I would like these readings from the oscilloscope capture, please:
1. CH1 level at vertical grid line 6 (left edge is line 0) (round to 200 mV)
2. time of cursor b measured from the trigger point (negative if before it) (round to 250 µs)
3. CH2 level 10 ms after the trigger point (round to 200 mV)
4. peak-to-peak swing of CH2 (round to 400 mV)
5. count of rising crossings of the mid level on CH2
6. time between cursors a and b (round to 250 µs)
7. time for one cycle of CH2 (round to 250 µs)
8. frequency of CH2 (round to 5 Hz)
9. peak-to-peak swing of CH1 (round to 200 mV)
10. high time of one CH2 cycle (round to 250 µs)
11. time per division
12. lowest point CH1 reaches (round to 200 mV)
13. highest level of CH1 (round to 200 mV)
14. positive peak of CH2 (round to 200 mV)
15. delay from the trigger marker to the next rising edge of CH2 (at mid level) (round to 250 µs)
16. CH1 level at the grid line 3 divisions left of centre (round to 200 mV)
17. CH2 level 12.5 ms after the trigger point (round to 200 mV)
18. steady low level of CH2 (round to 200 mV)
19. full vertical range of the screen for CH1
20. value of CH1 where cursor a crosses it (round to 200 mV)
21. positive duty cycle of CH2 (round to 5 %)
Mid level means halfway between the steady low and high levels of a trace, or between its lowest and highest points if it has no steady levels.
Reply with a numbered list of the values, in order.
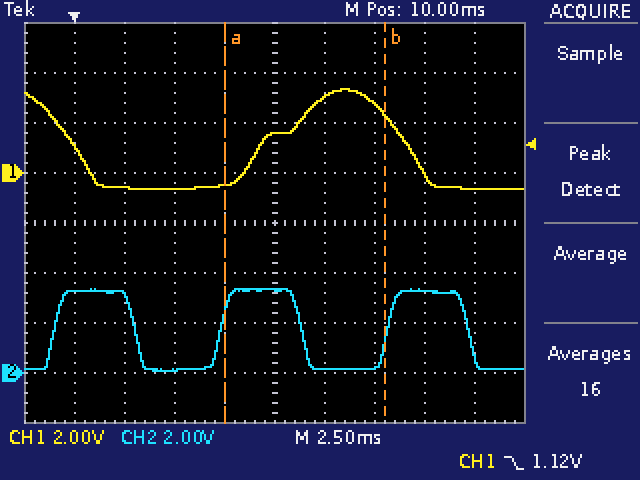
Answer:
1. 3.0 V
2. +15.50 ms
3. 3.4 V
4. 3.2 V
5. 3
6. 8.00 ms
7. 8.25 ms
8. 120 Hz
9. 4.0 V
10. 4.00 ms
11. 2.5 ms
12. -600 mV
13. 3.4 V
14. 3.4 V
15. 7.25 ms
16. -600 mV
17. 200 mV
18. 200 mV
19. 16 V
20. -400 mV
21. 50 %
